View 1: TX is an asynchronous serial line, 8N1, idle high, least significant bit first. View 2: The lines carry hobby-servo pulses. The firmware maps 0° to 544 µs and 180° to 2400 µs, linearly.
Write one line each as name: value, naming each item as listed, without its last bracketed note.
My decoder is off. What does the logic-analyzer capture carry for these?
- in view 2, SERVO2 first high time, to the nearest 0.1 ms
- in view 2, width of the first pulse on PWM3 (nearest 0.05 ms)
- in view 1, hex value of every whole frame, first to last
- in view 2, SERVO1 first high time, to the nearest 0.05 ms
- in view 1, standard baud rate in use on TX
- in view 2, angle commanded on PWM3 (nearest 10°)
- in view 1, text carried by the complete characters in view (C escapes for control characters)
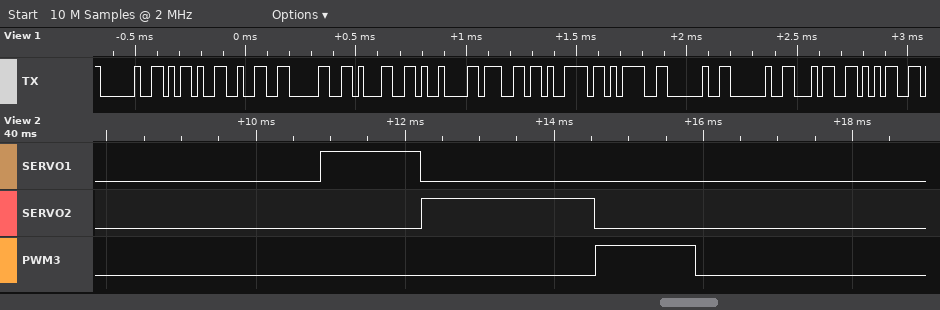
in view 2, SERVO2 first high time, to the nearest 0.1 ms: 2.3 ms
in view 2, width of the first pulse on PWM3: 1.35 ms
in view 1, hex value of every whole frame, first to last: 20 2D 32 30 31 09 67 79 3D 20 20 34 35
in view 2, SERVO1 first high time, to the nearest 0.05 ms: 1.35 ms
in view 1, standard baud rate in use on TX: 38400 baud
in view 2, angle commanded on PWM3: 80°
in view 1, text carried by the complete characters in view: " -201\tgy=  45"
